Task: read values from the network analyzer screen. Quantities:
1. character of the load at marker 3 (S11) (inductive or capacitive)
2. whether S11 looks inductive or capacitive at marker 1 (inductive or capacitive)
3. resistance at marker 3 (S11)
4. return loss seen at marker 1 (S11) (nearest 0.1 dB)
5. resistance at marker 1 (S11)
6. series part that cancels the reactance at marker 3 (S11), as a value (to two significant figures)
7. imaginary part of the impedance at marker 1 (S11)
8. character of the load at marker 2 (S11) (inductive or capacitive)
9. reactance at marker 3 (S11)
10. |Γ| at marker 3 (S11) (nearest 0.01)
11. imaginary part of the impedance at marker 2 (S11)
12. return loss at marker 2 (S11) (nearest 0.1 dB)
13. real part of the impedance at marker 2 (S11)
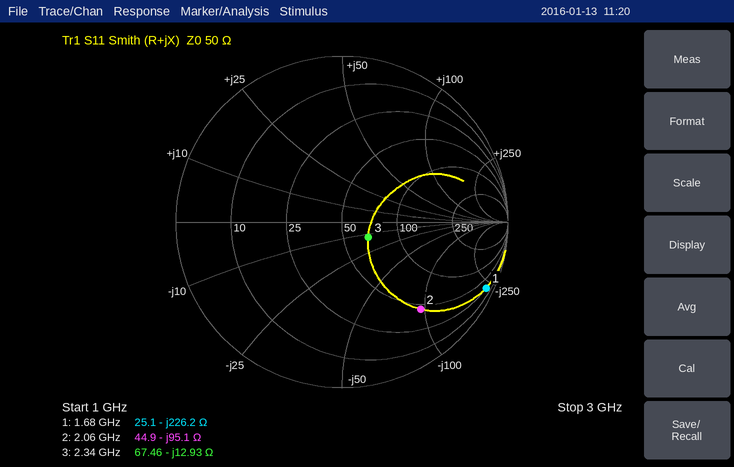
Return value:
capacitive
capacitive
67.46 Ω
0.4 dB
25.1 Ω
880 pH
-226.2 Ω
capacitive
-12.93 Ω
0.18
-95.1 Ω
3.0 dB
44.9 Ω
